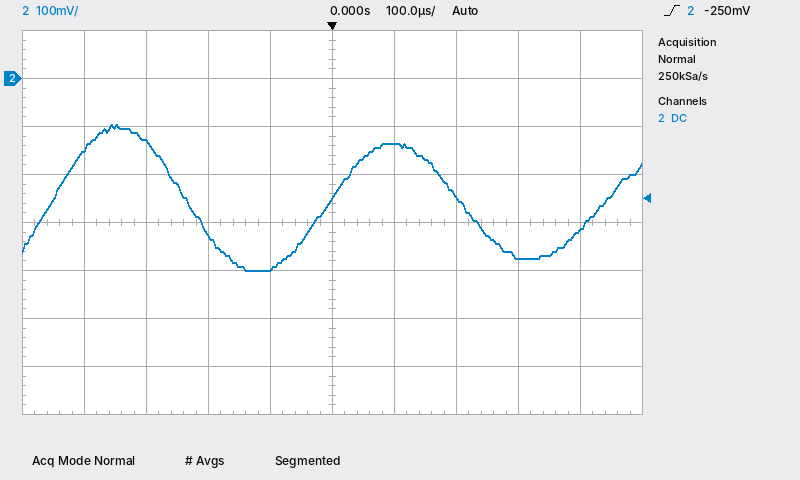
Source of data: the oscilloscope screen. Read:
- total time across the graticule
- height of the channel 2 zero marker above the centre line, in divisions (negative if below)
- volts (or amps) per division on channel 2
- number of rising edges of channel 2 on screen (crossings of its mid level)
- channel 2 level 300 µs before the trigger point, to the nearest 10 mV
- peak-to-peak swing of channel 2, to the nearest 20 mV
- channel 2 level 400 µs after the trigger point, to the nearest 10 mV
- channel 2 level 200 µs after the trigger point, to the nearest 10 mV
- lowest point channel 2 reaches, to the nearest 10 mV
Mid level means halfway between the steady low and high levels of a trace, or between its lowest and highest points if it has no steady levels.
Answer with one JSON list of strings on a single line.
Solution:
["1 ms", "+3.0 div", "100 mV", "3", "-130 mV", "300 mV", "-320 mV", "-250 mV", "-400 mV"]
